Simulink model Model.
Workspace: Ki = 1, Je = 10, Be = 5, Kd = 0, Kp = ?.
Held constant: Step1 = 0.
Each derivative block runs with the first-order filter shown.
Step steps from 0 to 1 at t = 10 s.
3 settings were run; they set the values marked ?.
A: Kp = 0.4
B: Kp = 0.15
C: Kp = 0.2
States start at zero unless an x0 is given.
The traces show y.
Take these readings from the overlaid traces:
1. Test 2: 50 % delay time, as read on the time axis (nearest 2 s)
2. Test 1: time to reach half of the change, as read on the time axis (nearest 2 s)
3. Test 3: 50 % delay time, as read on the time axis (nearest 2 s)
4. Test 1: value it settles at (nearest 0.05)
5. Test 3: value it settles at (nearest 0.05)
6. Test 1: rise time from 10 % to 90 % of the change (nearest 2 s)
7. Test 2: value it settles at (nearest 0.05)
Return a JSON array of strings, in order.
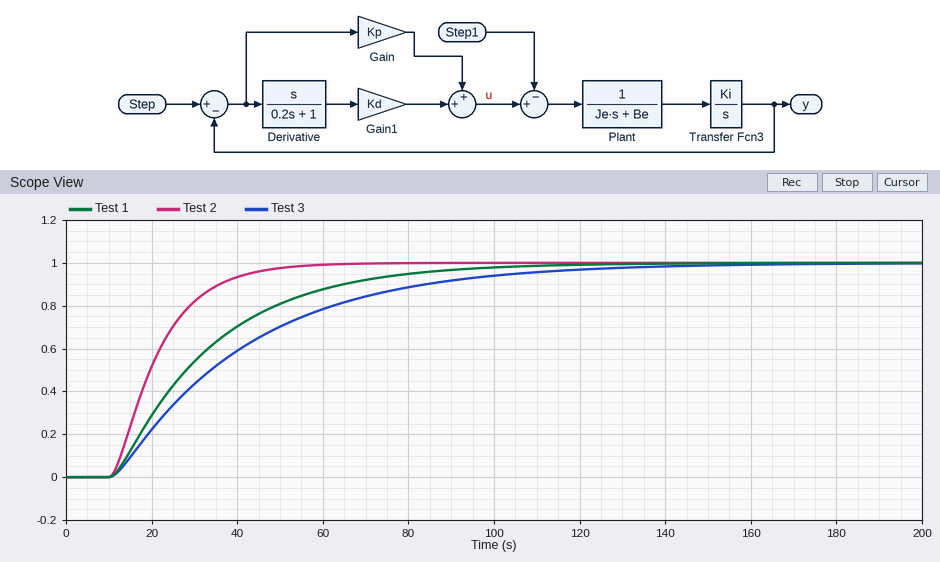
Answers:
["20 s", "28 s", "34 s", "1.00", "1.00", "50 s", "1.00"]
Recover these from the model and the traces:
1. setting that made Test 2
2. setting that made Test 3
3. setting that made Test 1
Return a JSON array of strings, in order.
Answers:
["A", "B", "C"]
